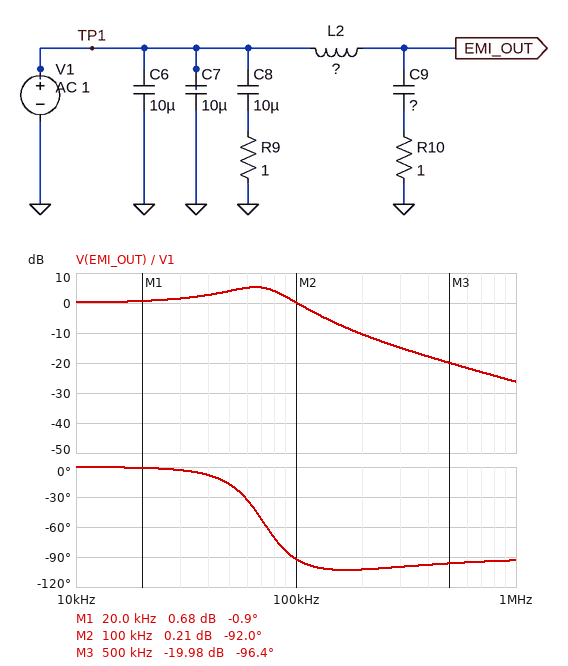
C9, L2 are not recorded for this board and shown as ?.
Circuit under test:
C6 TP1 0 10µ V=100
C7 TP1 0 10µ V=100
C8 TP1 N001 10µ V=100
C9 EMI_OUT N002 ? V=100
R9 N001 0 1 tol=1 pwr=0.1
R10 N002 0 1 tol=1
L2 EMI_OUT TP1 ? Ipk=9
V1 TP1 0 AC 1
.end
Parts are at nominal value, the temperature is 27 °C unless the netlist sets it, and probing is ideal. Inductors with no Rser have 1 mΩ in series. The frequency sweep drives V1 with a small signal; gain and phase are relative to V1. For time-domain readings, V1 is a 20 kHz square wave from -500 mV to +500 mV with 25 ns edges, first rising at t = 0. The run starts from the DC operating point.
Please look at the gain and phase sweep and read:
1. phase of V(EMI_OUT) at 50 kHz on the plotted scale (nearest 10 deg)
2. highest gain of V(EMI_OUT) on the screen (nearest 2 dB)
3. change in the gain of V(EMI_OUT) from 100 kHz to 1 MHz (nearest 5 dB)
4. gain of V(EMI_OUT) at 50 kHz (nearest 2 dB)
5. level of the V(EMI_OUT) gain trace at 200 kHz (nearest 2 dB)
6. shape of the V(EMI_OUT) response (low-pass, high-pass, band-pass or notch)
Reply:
-20 deg
6 dB
-25 dB
4 dB
-10 dB
low-pass
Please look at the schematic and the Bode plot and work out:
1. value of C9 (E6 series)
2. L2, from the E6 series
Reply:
1.5 µF
3.3 µH
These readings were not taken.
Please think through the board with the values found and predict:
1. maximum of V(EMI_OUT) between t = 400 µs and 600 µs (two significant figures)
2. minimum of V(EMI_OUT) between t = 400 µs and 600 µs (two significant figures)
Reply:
920 mV
-920 mV
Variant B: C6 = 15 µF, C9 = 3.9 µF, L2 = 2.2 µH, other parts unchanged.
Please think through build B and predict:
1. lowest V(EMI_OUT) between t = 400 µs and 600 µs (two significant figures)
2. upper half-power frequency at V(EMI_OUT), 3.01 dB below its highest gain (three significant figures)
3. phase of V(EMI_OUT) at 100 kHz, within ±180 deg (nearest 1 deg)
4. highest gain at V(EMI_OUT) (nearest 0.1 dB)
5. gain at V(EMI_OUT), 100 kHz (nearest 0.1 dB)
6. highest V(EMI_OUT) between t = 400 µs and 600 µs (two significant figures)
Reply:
-720 mV
84.3 kHz
-66 deg
2.3 dB
-2.2 dB
720 mV
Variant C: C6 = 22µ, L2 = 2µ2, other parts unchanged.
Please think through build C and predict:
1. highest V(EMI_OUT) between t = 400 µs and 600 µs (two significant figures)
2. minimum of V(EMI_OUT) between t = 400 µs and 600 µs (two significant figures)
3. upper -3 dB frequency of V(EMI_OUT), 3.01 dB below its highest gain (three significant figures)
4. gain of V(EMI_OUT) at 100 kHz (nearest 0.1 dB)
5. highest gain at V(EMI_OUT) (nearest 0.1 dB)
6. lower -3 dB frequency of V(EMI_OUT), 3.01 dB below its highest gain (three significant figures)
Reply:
850 mV
-850 mV
114 kHz
2.8 dB
4.2 dB
33.1 kHz
